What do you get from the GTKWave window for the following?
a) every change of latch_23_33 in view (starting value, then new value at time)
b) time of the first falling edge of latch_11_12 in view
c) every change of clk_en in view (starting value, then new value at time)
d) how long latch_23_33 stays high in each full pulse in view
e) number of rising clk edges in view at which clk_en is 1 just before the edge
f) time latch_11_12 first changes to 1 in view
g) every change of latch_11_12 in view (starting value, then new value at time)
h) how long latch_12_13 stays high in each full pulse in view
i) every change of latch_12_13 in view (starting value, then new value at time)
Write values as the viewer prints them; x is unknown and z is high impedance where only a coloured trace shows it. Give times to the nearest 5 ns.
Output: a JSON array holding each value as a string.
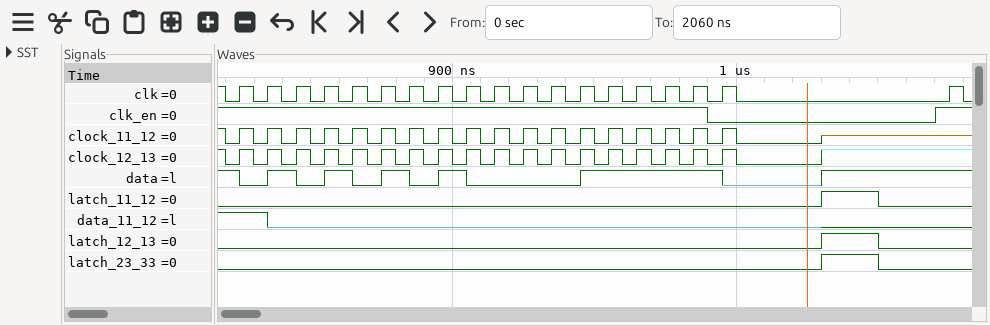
["0, 1 at 1030 ns, 0 at 1050 ns", "1050 ns", "1, 0 at 990 ns, 1 at 1070 ns", "20 ns", "18", "1030 ns", "0, 1 at 1030 ns, 0 at 1050 ns", "20 ns", "0, 1 at 1030 ns, 0 at 1050 ns"]
